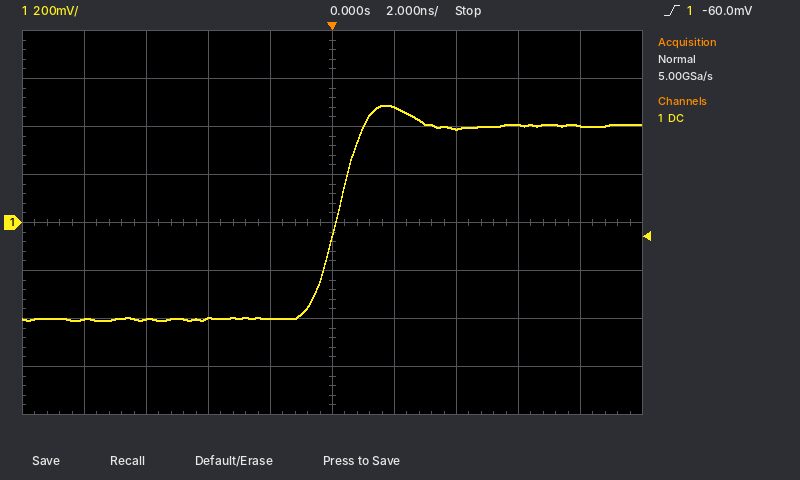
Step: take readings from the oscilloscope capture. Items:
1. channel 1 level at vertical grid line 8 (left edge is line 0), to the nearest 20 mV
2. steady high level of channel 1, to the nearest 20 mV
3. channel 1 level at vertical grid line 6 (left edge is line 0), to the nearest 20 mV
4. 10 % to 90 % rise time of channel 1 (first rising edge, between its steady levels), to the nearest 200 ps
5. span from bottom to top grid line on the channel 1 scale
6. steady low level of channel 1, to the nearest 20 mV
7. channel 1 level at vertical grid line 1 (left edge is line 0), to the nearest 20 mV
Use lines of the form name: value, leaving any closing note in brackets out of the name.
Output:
channel 1 level at vertical grid line 8 (left edge is line 0), to the nearest 20 mV: 400 mV
steady high level of channel 1, to the nearest 20 mV: 400 mV
channel 1 level at vertical grid line 6 (left edge is line 0), to the nearest 20 mV: 480 mV
10 % to 90 % rise time of channel 1 (first rising edge, between its steady levels), to the nearest 200 ps: 1.4 ns
span from bottom to top grid line on the channel 1 scale: 1.6 V
steady low level of channel 1, to the nearest 20 mV: -400 mV
channel 1 level at vertical grid line 1 (left edge is line 0), to the nearest 20 mV: -400 mV
